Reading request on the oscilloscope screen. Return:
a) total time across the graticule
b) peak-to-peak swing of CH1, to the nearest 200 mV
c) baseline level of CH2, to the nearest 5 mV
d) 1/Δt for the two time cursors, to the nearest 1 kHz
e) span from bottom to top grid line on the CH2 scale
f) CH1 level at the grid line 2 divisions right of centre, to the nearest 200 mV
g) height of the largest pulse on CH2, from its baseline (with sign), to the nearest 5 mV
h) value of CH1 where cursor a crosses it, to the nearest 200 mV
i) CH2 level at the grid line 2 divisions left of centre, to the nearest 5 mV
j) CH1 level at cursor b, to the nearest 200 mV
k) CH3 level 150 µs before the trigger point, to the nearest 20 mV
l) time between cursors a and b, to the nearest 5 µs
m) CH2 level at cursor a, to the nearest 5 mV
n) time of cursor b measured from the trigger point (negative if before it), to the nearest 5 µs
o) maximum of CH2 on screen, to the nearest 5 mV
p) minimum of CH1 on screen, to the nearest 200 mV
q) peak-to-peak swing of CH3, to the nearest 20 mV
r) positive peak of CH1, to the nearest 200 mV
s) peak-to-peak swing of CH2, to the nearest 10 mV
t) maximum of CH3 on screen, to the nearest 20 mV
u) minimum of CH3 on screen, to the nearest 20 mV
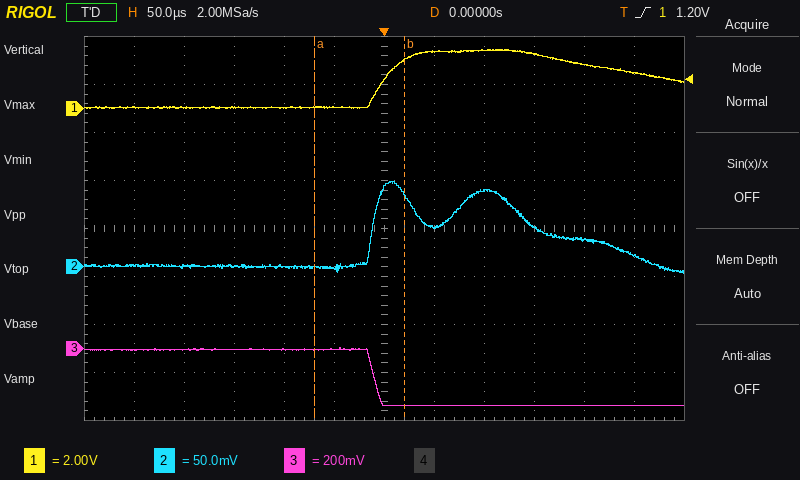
600 µs
2.4 V
0 mV
11 kHz
400 mV
2.4 V
+90 mV
0.0 V
0 mV
2.0 V
0 mV
90 µs
0 mV
+20 µs
90 mV
0.0 V
240 mV
2.4 V
100 mV
0 mV
-240 mV
